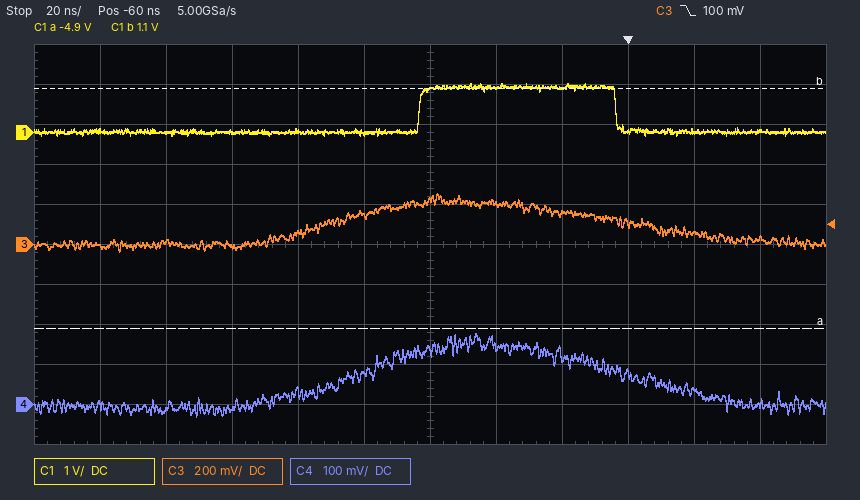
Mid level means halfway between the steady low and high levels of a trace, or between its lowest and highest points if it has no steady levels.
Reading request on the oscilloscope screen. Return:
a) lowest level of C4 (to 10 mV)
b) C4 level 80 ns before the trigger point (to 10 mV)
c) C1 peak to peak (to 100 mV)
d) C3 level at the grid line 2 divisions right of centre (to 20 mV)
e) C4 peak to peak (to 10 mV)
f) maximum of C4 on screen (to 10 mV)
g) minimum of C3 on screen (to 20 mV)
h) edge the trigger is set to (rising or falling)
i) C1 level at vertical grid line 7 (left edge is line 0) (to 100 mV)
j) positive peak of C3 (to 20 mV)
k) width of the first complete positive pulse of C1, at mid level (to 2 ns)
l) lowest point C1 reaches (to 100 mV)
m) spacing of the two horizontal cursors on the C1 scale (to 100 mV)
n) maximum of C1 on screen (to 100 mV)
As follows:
-30 mV
80 mV
1.3 V
160 mV
210 mV
180 mV
-40 mV
falling
1.1 V
260 mV
60 ns
-100 mV
6.0 V
1.2 V
